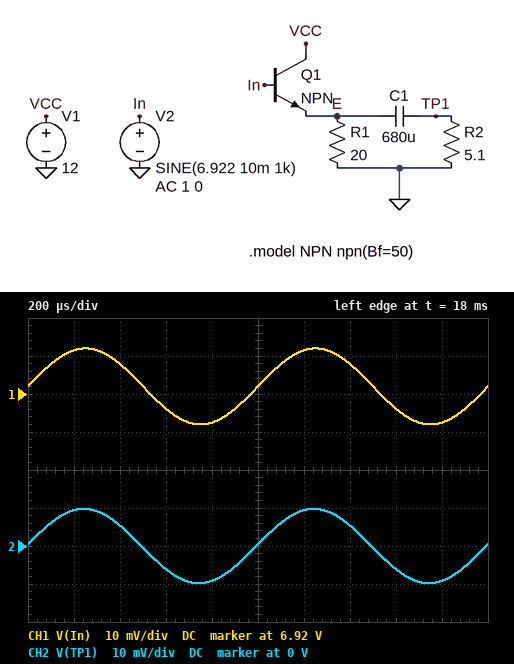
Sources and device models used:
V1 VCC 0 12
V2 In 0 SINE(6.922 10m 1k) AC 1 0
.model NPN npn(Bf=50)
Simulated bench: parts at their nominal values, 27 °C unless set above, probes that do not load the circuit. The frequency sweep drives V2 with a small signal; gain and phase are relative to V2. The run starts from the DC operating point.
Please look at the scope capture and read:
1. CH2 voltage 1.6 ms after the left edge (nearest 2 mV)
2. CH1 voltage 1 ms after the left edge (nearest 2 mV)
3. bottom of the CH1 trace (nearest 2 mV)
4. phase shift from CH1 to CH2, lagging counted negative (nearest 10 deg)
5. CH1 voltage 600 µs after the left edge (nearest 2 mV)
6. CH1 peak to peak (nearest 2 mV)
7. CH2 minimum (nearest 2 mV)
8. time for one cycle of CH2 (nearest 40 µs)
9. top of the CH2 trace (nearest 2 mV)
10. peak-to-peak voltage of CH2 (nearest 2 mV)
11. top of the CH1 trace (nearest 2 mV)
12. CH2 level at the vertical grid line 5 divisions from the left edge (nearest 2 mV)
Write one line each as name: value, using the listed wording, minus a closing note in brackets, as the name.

CH2 voltage 1.6 ms after the left edge: -6 mV
CH1 voltage 1 ms after the left edge: 6.922 V
bottom of the CH1 trace: 6.912 V
phase shift from CH1 to CH2, lagging counted negative: 0 deg
CH1 voltage 600 µs after the left edge: 6.916 V
CH1 peak to peak: 20 mV
CH2 minimum: -10 mV
time for one cycle of CH2: 1.00 ms
top of the CH2 trace: 10 mV
peak-to-peak voltage of CH2: 20 mV
top of the CH1 trace: 6.932 V
CH2 level at the vertical grid line 5 divisions from the left edge: 0 V
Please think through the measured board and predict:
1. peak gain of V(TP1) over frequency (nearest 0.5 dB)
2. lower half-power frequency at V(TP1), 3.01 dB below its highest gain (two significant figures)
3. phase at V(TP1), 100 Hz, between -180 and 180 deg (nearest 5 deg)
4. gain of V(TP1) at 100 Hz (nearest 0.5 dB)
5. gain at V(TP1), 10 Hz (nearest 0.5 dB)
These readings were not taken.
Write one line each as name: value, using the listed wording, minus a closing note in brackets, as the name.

peak gain of V(TP1) over frequency: 0 dB
lower half-power frequency at V(TP1), 3.01 dB below its highest gain: 45 Hz
phase at V(TP1), 100 Hz, between -180 and 180 deg: 25 deg
gain of V(TP1) at 100 Hz: -1.0 dB
gain at V(TP1), 10 Hz: -13.5 dB
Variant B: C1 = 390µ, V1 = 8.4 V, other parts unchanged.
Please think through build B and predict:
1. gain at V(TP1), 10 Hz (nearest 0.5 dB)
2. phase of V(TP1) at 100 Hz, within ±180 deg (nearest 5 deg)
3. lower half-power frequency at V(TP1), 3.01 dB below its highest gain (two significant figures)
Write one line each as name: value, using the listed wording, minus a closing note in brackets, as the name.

gain at V(TP1), 10 Hz: -18.0 dB
phase of V(TP1) at 100 Hz, within ±180 deg: 40 deg
lower half-power frequency at V(TP1), 3.01 dB below its highest gain: 79 Hz
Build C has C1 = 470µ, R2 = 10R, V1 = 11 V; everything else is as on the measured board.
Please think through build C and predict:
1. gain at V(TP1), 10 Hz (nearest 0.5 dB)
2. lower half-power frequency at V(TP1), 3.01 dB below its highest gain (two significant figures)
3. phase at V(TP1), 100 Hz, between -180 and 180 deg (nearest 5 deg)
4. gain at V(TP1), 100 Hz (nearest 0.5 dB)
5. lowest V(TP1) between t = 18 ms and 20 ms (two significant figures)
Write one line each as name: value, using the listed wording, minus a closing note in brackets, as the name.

gain at V(TP1), 10 Hz: -11.0 dB
lower half-power frequency at V(TP1), 3.01 dB below its highest gain: 34 Hz
phase at V(TP1), 100 Hz, between -180 and 180 deg: 20 deg
gain at V(TP1), 100 Hz: -0.5 dB
lowest V(TP1) between t = 18 ms and 20 ms: -9.9 mV
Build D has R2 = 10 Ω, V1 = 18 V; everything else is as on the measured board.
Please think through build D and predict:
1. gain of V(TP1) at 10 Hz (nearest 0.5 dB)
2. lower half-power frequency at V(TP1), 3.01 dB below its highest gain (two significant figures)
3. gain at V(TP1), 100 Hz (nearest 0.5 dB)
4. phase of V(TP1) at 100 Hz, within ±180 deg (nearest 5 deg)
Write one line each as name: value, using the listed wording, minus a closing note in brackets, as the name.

gain of V(TP1) at 10 Hz: -8.0 dB
lower half-power frequency at V(TP1), 3.01 dB below its highest gain: 23 Hz
gain at V(TP1), 100 Hz: -0.5 dB
phase of V(TP1) at 100 Hz, within ±180 deg: 15 deg
